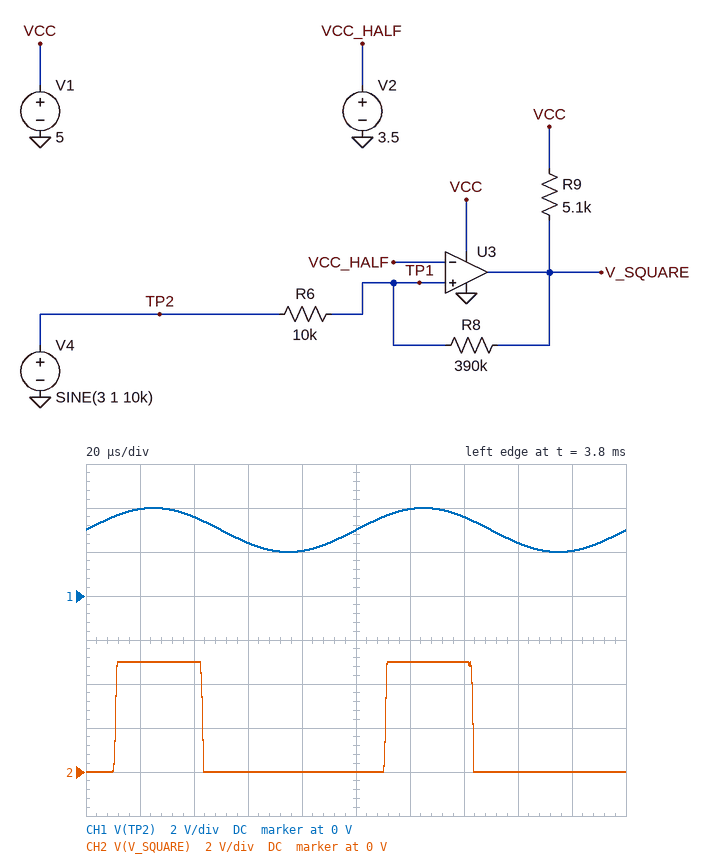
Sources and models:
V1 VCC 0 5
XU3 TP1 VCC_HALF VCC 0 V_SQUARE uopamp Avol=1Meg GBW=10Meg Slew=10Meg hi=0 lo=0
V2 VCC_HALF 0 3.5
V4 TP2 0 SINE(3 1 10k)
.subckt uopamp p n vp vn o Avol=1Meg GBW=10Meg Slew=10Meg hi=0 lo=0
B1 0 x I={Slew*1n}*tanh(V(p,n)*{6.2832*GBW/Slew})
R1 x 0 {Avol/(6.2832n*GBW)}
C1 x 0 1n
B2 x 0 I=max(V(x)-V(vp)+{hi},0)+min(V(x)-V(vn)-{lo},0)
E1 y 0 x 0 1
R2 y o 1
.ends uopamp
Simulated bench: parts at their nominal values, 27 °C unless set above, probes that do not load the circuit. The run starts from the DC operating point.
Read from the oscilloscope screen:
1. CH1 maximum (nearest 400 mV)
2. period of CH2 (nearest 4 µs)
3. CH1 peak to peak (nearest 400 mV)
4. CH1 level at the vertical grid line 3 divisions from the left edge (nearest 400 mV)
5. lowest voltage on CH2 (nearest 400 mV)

4.0 V
100 µs
2.0 V
2.4 V
0 V
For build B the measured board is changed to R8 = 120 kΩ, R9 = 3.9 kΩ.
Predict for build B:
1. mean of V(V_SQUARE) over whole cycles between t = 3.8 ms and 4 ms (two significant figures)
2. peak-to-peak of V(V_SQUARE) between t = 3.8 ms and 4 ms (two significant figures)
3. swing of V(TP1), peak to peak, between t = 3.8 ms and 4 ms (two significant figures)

1.5 V
5.0 V
2.2 V
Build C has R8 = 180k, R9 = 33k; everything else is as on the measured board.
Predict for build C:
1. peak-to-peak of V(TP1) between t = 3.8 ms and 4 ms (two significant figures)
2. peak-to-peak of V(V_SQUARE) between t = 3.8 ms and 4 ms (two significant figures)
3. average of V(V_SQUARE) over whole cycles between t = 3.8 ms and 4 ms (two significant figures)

2.2 V
5.0 V
1.5 V
